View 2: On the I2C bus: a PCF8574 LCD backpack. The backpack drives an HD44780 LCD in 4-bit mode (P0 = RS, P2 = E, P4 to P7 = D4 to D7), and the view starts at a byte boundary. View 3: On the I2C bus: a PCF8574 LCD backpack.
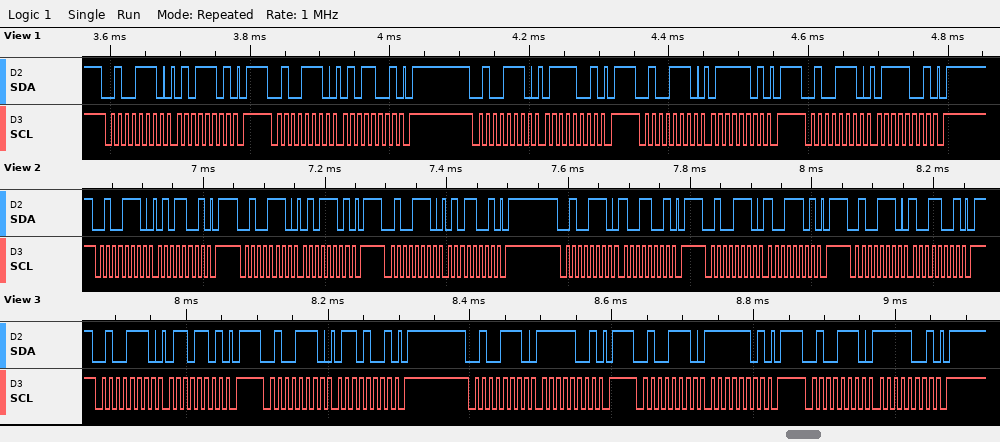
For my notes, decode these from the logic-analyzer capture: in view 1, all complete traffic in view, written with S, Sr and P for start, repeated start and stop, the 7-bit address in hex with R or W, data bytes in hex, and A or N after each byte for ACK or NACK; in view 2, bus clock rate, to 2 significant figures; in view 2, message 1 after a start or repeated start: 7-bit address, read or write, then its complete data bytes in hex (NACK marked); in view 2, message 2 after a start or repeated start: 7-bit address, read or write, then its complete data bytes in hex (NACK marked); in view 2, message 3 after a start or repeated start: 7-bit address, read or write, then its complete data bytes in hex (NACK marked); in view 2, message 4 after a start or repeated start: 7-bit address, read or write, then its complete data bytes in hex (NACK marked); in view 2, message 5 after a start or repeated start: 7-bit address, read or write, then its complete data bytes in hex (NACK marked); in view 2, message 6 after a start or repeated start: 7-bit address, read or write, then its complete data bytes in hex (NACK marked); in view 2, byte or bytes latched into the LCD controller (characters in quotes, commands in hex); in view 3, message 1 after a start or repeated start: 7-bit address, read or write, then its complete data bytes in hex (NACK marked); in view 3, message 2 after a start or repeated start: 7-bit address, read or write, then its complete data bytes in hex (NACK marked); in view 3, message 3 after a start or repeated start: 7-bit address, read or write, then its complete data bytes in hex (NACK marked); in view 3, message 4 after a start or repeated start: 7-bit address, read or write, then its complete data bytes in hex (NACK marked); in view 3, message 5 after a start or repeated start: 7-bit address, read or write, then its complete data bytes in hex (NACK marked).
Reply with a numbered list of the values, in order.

1. S 27W A 5D A P S 27W A 59 A P S 27W A 79 A P S 27W A 7D A P S 27W A 79 A P
2. 100 kHz
3. 0x27 write: 59
4. 0x27 write: 5D
5. 0x27 write: 59
6. 0x27 write: 99
7. 0x27 write: 9D
8. 0x27 write: 99
9. 'Y'
10. 0x27 write: 6D
11. 0x27 write: 69
12. 0x27 write: F9
13. 0x27 write: FD
14. 0x27 write: F9
